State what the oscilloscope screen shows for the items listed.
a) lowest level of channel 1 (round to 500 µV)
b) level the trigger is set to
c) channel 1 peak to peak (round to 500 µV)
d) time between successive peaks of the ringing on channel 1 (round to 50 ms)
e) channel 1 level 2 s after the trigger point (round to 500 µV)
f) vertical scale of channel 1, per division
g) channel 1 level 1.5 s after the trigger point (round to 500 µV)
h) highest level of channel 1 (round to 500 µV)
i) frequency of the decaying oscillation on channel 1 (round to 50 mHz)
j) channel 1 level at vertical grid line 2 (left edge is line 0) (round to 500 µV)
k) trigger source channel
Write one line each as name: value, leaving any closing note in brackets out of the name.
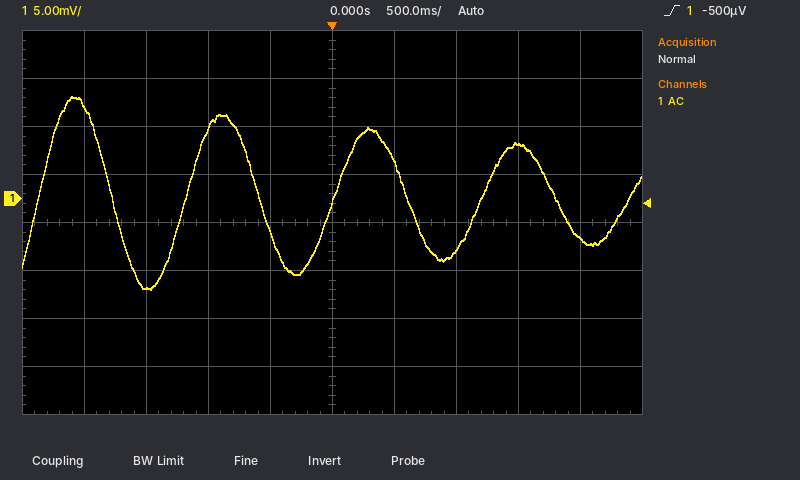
lowest level of channel 1: -9.5 mV
level the trigger is set to: -500 µV
channel 1 peak to peak: 20.0 mV
time between successive peaks of the ringing on channel 1: 1.20 s
channel 1 level 2 s after the trigger point: -4.0 mV
vertical scale of channel 1, per division: 5 mV
channel 1 level 1.5 s after the trigger point: 5.5 mV
highest level of channel 1: 10.5 mV
frequency of the decaying oscillation on channel 1: 850 mHz
channel 1 level at vertical grid line 2 (left edge is line 0): -9.5 mV
trigger source channel: channel 1
